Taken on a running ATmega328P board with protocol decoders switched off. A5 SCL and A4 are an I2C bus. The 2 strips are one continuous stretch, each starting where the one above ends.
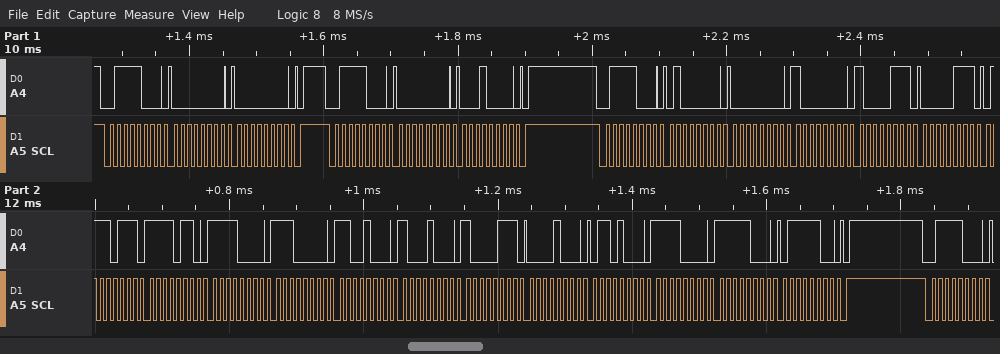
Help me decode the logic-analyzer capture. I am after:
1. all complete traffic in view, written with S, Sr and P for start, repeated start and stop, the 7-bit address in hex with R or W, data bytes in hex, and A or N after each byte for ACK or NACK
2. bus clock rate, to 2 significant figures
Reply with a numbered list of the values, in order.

1. S 3CW A 00 A 00 A P S 3CW A 00 A 10 A P S 3CW A 40 A 00 A 80 A 87 A 07 A 77 A F6 A F0 A E0 A C8 A 88 A 87 A 08 A 68 A F0 A F8 A 7C A P S 3CW A
2. 100 kHz
